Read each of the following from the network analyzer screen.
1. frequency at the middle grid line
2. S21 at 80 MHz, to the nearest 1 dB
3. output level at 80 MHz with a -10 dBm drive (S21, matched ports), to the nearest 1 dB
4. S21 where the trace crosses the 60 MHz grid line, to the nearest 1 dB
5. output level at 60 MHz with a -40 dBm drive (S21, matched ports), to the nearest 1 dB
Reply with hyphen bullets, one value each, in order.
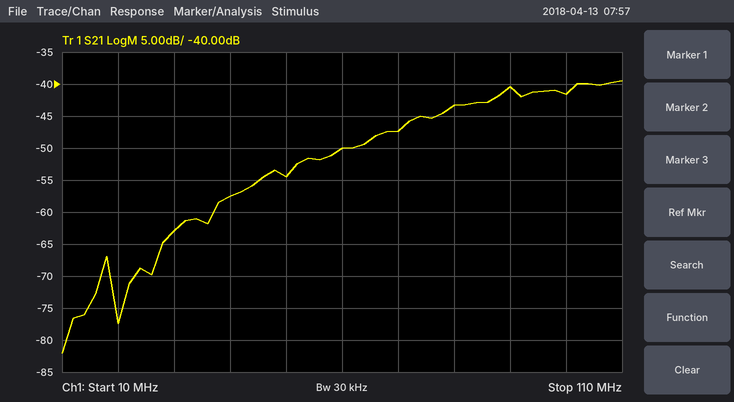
- 60 MHz
- -43 dB
- -53 dBm
- -50 dB
- -90 dBm
